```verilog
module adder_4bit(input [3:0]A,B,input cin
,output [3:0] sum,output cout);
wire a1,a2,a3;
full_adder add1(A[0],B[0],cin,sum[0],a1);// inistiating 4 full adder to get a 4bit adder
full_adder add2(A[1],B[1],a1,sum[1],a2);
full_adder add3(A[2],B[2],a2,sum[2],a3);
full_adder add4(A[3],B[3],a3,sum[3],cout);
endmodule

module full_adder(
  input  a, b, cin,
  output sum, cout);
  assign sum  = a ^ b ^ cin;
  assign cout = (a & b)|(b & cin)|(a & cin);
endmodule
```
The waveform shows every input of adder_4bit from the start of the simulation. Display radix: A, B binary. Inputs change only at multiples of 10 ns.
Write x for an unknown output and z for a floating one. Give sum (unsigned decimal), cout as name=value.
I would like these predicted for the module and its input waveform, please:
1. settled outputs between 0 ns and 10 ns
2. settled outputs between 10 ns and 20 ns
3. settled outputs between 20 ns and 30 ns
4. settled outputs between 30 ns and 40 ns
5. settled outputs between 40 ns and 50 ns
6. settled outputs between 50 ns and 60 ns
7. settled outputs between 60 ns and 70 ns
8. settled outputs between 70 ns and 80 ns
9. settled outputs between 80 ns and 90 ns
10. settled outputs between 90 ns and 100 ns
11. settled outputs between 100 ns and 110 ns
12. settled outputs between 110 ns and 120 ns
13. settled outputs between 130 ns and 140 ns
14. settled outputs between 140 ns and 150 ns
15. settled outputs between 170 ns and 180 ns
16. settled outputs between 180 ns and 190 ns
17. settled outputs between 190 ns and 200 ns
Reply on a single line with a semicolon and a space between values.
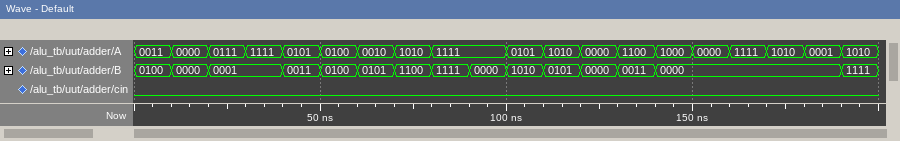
sum=7, cout=0; sum=0, cout=0; sum=8, cout=0; sum=0, cout=1; sum=8, cout=0; sum=8, cout=0; sum=7, cout=0; sum=6, cout=1; sum=14, cout=1; sum=15, cout=0; sum=15, cout=0; sum=15, cout=0; sum=15, cout=0; sum=8, cout=0; sum=10, cout=0; sum=1, cout=0; sum=9, cout=1
